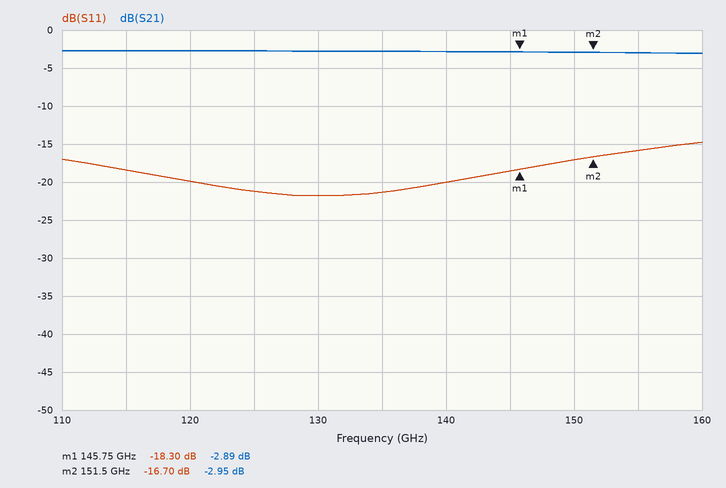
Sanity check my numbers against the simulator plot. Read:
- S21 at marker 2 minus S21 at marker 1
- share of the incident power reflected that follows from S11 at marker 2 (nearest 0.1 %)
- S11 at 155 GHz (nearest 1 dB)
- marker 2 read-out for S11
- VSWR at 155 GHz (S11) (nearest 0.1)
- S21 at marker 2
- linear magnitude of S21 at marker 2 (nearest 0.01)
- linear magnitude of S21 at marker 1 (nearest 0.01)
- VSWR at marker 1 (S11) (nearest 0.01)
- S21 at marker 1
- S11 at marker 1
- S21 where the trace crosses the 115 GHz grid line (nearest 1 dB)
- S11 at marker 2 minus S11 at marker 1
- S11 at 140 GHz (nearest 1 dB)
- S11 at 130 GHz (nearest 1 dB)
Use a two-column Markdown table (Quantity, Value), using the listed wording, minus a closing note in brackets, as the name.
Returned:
| Quantity | Value |
|---|---|
| S21 at marker 2 minus S21 at marker 1 | -0.06 dB |
| share of the incident power reflected that follows from S11 at marker 2 | 2.1 % |
| S11 at 155 GHz | -16 dB |
| marker 2 read-out for S11 | -16.70 dB |
| VSWR at 155 GHz (S11) | 1.4 |
| S21 at marker 2 | -2.95 dB |
| linear magnitude of S21 at marker 2 | 0.71 |
| linear magnitude of S21 at marker 1 | 0.72 |
| VSWR at marker 1 (S11) | 1.28 |
| S21 at marker 1 | -2.89 dB |
| S11 at marker 1 | -18.30 dB |
| S21 where the trace crosses the 115 GHz grid line | -3 dB |
| S11 at marker 2 minus S11 at marker 1 | 1.60 dB |
| S11 at 140 GHz | -20 dB |
| S11 at 130 GHz | -22 dB |
